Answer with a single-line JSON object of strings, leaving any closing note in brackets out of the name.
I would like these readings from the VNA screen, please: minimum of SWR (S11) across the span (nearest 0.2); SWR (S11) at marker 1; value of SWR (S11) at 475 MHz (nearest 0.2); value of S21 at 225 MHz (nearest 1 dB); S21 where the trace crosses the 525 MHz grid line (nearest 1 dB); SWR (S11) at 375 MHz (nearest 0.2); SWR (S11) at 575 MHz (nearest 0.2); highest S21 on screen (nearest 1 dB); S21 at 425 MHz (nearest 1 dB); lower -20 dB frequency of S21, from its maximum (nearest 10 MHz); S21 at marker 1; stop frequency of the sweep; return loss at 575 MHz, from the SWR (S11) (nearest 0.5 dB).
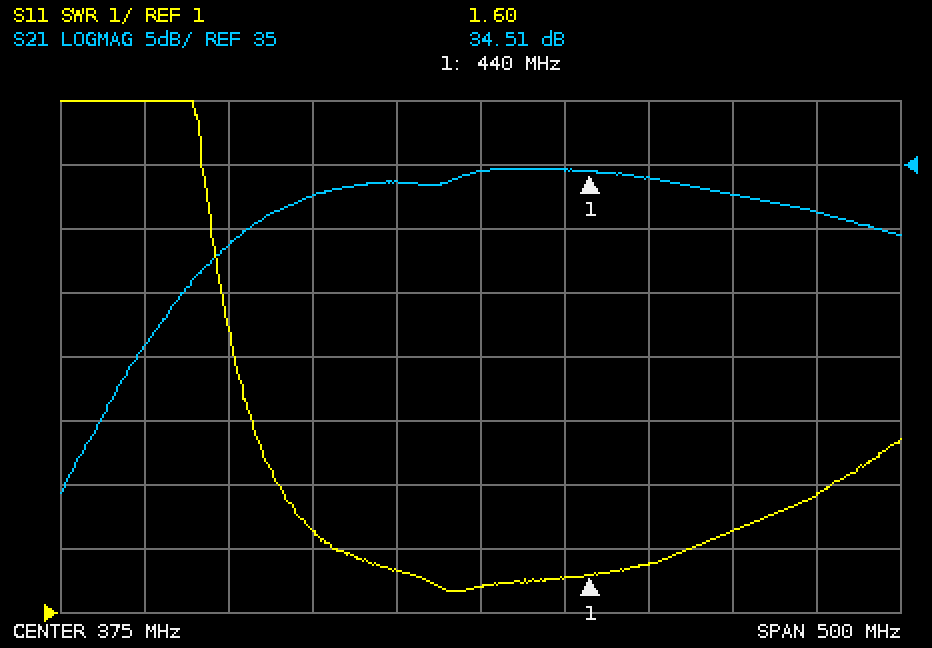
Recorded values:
{"minimum of SWR (S11) across the span": "1.4", "SWR (S11) at marker 1": "1.60", "value of SWR (S11) at 475 MHz": "1.8", "value of S21 at 225 MHz": "29 dB", "S21 where the trace crosses the 525 MHz grid line": "33 dB", "SWR (S11) at 375 MHz": "1.4", "SWR (S11) at 575 MHz": "2.8", "highest S21 on screen": "35 dB", "S21 at 425 MHz": "35 dB", "lower -20 dB frequency of S21, from its maximum": "150 MHz", "S21 at marker 1": "34.51 dB", "stop frequency of the sweep": "625 MHz", "return loss at 575 MHz, from the SWR (S11)": "6.5 dB"}
